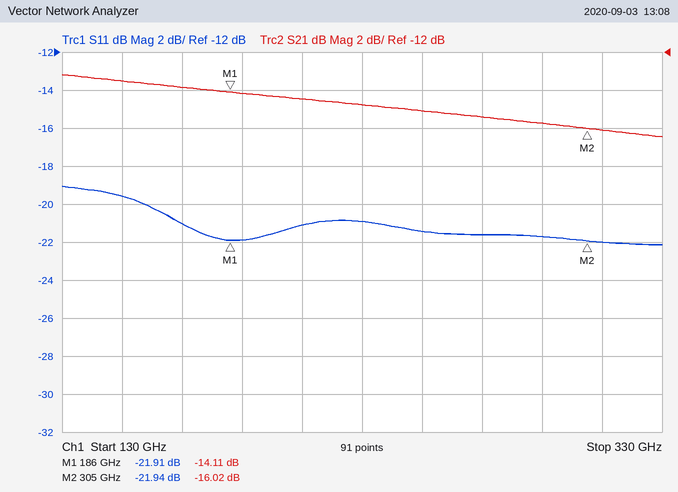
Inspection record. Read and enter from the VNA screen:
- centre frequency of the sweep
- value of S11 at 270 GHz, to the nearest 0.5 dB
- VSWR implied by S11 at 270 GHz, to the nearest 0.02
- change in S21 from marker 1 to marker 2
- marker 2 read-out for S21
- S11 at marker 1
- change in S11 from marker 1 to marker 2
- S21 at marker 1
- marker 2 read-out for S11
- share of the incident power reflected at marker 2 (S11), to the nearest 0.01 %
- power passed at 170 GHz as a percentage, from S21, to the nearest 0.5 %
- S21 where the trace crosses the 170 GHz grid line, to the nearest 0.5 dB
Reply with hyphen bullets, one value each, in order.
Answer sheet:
- 230 GHz
- -21.5 dB
- 1.18
- -1.91 dB
- -16.02 dB
- -21.91 dB
- -0.03 dB
- -14.11 dB
- -21.94 dB
- 0.64 %
- 4.0 %
- -14.0 dB
